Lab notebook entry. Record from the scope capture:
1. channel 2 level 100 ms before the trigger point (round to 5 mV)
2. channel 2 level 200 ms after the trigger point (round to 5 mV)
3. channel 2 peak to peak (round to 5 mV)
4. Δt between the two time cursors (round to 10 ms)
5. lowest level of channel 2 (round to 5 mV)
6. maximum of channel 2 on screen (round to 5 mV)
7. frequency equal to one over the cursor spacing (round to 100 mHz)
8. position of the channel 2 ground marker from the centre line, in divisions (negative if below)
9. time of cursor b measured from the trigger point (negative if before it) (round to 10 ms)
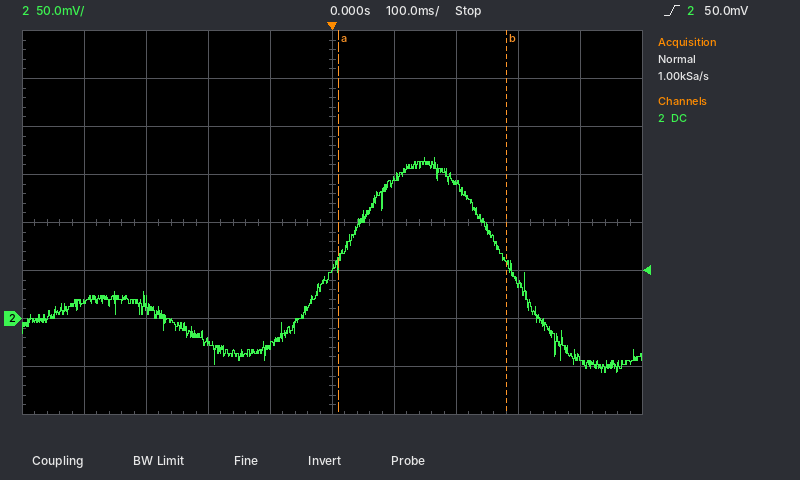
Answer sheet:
-30 mV
140 mV
225 mV
270 ms
-55 mV
170 mV
3.7 Hz
-2.0 div
+280 ms
